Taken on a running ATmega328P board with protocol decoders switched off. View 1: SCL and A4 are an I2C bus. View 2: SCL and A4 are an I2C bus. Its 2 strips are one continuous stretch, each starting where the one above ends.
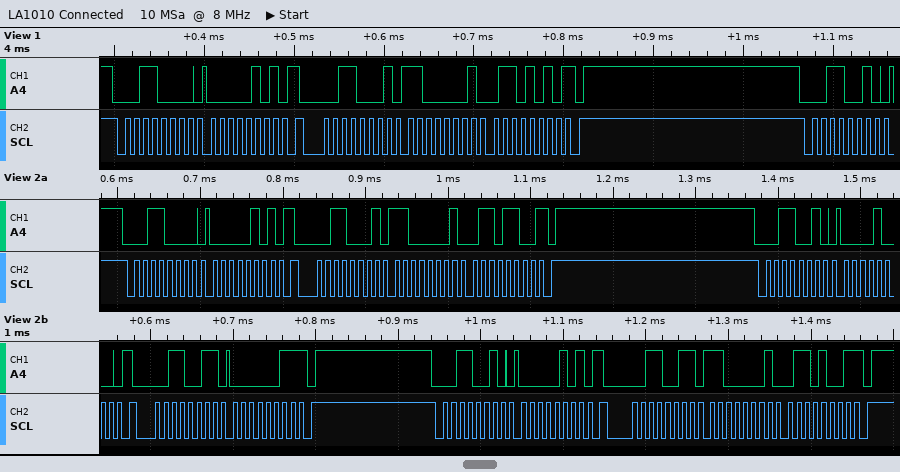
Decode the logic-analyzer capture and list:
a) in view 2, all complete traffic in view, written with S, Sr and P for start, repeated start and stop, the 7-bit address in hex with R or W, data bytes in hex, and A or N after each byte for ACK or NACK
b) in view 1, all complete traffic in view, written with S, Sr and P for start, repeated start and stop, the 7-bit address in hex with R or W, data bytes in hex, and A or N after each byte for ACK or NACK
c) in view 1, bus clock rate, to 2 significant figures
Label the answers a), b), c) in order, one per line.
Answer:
a) S 18W A 05 A Sr 18R A C1 A 6C N P S 19W A 08 A Sr 19R A 03 N P S 19W A 05 A Sr 19R A C1 A 69 N P
b) S 18W A 05 A Sr 18R A C1 A 6A N P S 19W A
c) 100 kHz
